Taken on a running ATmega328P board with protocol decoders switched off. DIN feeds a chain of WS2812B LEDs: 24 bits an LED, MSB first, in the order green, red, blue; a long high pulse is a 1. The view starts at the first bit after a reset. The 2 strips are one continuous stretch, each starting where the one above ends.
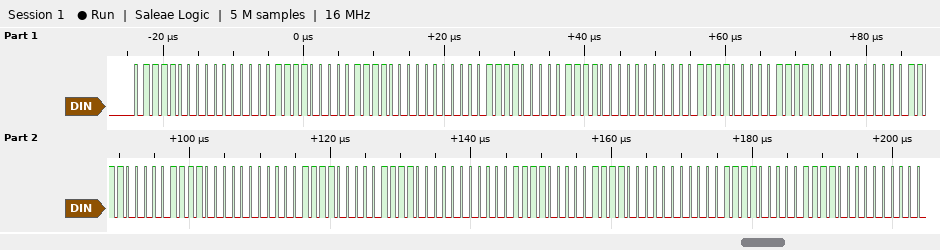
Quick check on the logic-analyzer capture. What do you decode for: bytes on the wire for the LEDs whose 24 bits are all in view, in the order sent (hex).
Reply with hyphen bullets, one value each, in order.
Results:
- 78 00 F0 78 00 F0 78 00 F0 78 00 F0 78 00 F0 78 00 F0 78 00 F0
